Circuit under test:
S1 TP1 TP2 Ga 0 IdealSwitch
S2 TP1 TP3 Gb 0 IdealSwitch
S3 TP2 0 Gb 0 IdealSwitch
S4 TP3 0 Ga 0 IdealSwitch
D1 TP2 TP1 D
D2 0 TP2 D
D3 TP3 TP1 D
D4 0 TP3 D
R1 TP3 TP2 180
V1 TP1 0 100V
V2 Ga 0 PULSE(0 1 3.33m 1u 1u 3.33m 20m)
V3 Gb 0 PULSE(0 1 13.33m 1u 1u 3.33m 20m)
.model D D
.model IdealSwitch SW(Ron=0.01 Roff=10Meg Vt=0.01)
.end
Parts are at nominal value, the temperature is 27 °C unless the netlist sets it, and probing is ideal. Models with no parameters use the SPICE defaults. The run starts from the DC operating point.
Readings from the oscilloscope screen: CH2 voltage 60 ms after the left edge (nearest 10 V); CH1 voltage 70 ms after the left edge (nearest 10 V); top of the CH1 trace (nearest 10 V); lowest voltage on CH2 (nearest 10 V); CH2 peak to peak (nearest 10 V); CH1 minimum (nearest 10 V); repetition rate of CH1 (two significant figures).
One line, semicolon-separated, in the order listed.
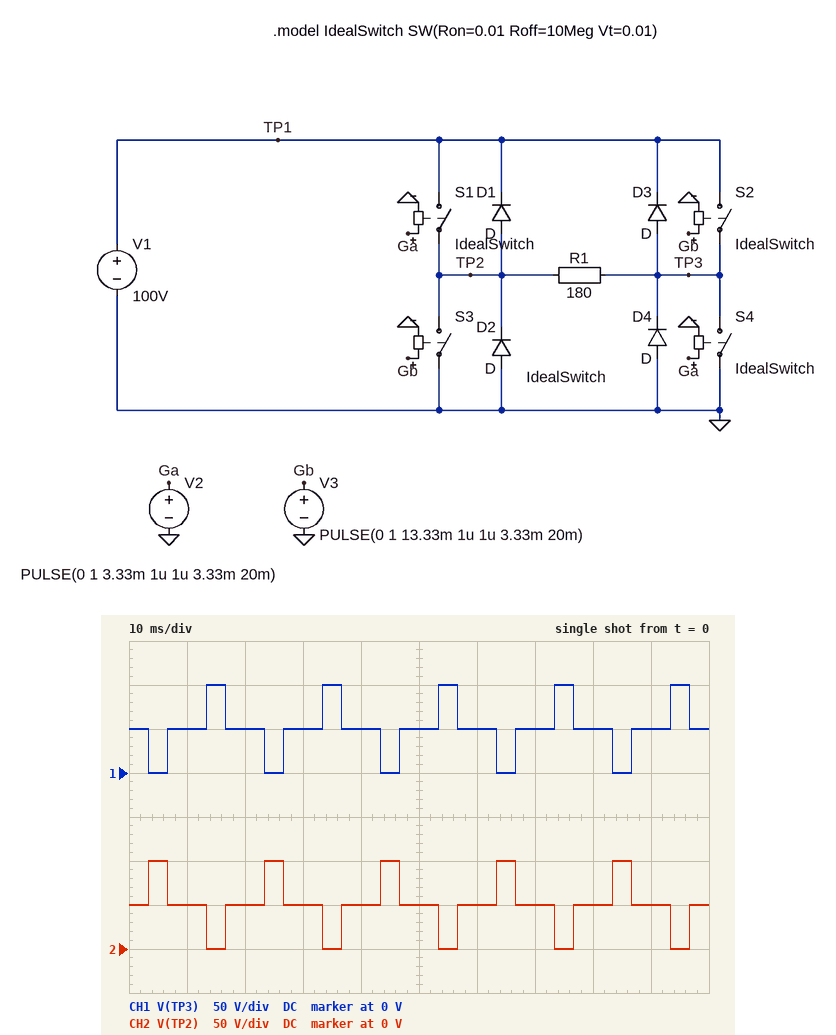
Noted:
50 V; 50 V; 100 V; 0 V; 100 V; 0 V; 50 Hz
